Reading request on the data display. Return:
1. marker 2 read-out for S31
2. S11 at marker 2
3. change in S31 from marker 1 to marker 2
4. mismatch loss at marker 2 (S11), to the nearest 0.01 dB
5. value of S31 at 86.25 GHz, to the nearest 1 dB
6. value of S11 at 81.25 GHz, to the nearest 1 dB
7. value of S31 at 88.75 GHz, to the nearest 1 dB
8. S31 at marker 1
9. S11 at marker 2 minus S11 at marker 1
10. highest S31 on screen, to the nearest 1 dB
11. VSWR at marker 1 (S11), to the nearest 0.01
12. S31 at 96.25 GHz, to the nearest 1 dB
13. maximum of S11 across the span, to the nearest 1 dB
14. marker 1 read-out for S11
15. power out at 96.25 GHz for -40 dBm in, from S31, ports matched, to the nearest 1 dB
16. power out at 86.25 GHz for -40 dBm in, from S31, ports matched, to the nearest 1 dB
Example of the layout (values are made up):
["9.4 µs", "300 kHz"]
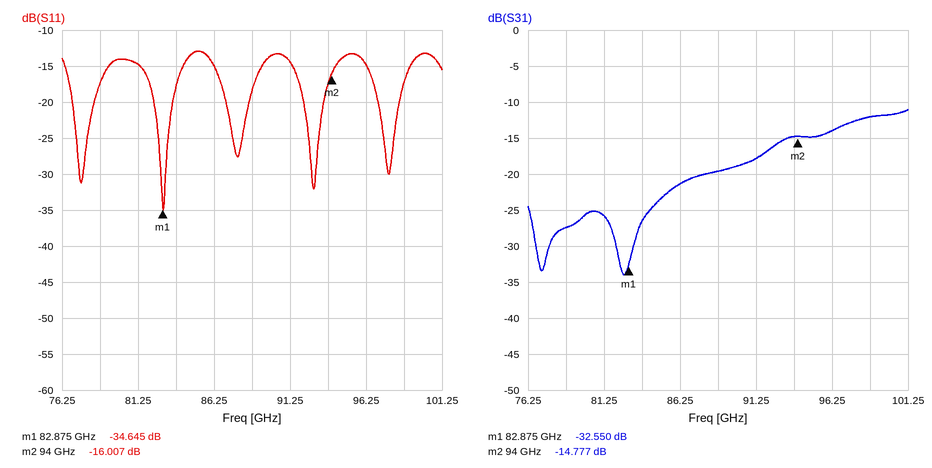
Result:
["-14.777 dB", "-16.007 dB", "17.773 dB", "0.11 dB", "-21 dB", "-15 dB", "-20 dB", "-32.550 dB", "18.638 dB", "-11 dB", "1.04", "-14 dB", "-13 dB", "-34.645 dB", "-54 dBm", "-61 dBm"]
